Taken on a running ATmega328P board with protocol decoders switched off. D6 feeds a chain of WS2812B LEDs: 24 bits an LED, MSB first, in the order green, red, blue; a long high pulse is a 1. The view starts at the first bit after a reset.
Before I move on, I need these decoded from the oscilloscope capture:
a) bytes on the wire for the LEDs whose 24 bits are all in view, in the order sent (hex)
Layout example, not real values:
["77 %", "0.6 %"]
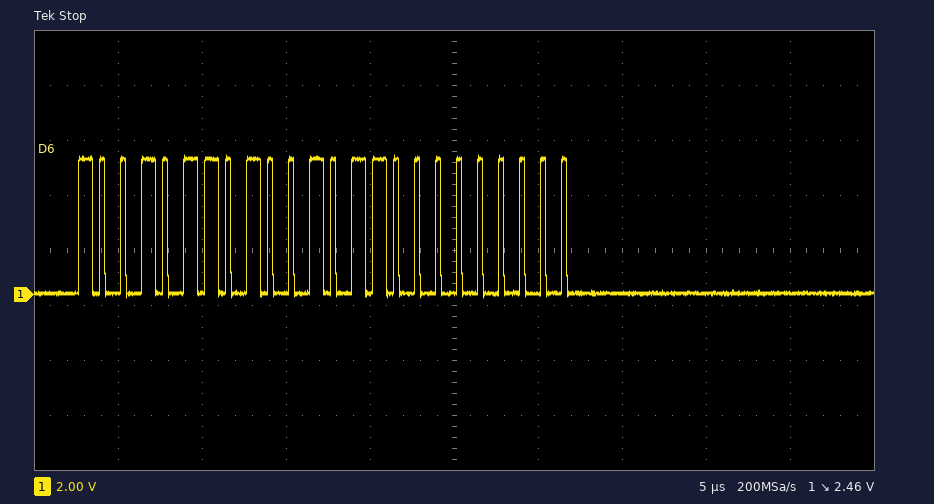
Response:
["96 96 00"]
